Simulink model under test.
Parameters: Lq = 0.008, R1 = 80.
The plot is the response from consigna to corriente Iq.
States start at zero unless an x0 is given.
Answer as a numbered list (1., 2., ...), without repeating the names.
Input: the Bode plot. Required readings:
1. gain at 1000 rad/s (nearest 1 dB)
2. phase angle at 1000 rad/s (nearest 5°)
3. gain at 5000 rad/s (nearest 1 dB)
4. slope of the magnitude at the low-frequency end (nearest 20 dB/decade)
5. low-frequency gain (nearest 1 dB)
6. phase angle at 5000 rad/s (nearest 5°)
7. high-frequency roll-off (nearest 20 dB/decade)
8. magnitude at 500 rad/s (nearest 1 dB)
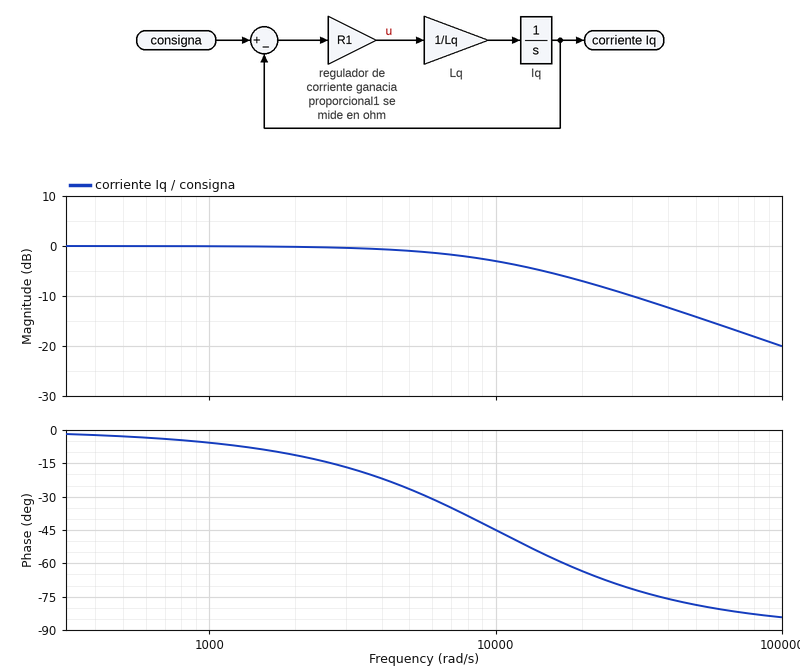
1. 0 dB
2. -5°
3. -1 dB
4. 0 dB/decade
5. 0 dB
6. -25°
7. -20 dB/decade
8. 0 dB
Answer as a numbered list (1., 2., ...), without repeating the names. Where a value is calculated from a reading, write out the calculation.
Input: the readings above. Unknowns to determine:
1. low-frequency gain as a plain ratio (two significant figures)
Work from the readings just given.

1. 10^(0 / 20) = 1.0
